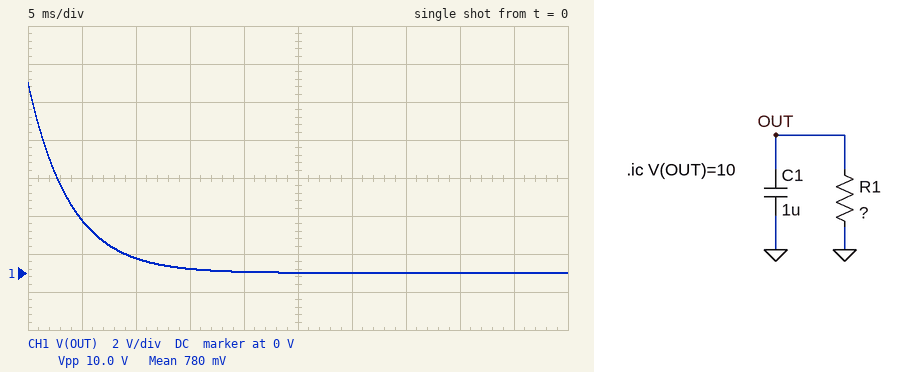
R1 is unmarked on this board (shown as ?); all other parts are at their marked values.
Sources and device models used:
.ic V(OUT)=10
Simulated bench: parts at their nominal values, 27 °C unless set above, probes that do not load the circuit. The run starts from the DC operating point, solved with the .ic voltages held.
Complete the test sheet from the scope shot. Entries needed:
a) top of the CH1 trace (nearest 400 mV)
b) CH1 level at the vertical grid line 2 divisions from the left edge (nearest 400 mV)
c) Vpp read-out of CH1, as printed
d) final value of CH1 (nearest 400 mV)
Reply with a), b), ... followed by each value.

a) 10.0 V
b) 800 mV
c) 10.0 V
d) 0 V
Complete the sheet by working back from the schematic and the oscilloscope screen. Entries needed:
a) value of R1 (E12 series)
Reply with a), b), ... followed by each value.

a) 3.9 kΩ
